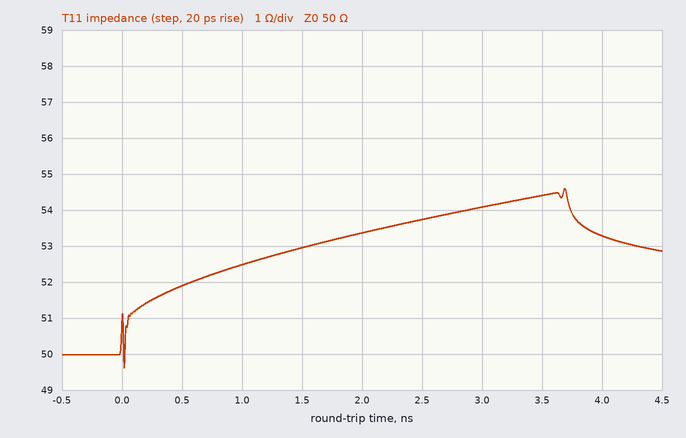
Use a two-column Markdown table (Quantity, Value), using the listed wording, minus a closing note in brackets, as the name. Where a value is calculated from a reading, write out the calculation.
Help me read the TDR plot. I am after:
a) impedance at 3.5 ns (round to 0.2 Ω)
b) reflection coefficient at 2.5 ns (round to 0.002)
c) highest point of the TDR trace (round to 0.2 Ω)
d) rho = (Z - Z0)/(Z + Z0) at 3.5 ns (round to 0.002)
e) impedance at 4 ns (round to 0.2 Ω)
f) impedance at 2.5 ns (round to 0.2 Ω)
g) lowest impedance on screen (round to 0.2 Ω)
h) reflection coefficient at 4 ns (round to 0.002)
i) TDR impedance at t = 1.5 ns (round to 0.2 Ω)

| Quantity | Value |
|---|---|
| impedance at 3.5 ns | 54.4 Ω |
| reflection coefficient at 2.5 ns | (53.8 − 50)/(53.8 + 50) ≈ +0.0366, so +0.036 to the nearest 0.002 |
| highest point of the TDR trace | 54.6 Ω |
| rho = (Z - Z0)/(Z + Z0) at 3.5 ns | (54.4 − 50)/(54.4 + 50) ≈ +0.042 |
| impedance at 4 ns | 53.2 Ω |
| impedance at 2.5 ns | 53.8 Ω |
| lowest impedance on screen | 49.6 Ω |
| reflection coefficient at 4 ns | (53.2 − 50)/(53.2 + 50) ≈ +0.0310, so +0.032 to the nearest 0.002 |
| TDR impedance at t = 1.5 ns | 53.0 Ω |
